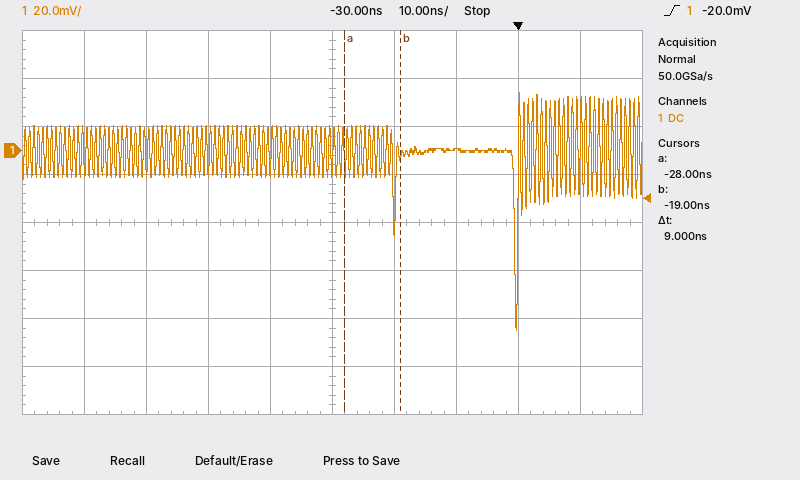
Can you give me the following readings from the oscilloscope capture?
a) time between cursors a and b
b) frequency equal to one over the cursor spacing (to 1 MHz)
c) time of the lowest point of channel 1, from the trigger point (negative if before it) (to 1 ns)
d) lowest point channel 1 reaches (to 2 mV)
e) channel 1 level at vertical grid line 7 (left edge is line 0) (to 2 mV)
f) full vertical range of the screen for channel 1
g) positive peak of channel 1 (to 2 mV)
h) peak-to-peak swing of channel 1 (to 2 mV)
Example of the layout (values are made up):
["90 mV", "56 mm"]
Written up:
["9 ns", "111 MHz", "0 ns", "-76 mV", "0 mV", "160 mV", "24 mV", "100 mV"]
